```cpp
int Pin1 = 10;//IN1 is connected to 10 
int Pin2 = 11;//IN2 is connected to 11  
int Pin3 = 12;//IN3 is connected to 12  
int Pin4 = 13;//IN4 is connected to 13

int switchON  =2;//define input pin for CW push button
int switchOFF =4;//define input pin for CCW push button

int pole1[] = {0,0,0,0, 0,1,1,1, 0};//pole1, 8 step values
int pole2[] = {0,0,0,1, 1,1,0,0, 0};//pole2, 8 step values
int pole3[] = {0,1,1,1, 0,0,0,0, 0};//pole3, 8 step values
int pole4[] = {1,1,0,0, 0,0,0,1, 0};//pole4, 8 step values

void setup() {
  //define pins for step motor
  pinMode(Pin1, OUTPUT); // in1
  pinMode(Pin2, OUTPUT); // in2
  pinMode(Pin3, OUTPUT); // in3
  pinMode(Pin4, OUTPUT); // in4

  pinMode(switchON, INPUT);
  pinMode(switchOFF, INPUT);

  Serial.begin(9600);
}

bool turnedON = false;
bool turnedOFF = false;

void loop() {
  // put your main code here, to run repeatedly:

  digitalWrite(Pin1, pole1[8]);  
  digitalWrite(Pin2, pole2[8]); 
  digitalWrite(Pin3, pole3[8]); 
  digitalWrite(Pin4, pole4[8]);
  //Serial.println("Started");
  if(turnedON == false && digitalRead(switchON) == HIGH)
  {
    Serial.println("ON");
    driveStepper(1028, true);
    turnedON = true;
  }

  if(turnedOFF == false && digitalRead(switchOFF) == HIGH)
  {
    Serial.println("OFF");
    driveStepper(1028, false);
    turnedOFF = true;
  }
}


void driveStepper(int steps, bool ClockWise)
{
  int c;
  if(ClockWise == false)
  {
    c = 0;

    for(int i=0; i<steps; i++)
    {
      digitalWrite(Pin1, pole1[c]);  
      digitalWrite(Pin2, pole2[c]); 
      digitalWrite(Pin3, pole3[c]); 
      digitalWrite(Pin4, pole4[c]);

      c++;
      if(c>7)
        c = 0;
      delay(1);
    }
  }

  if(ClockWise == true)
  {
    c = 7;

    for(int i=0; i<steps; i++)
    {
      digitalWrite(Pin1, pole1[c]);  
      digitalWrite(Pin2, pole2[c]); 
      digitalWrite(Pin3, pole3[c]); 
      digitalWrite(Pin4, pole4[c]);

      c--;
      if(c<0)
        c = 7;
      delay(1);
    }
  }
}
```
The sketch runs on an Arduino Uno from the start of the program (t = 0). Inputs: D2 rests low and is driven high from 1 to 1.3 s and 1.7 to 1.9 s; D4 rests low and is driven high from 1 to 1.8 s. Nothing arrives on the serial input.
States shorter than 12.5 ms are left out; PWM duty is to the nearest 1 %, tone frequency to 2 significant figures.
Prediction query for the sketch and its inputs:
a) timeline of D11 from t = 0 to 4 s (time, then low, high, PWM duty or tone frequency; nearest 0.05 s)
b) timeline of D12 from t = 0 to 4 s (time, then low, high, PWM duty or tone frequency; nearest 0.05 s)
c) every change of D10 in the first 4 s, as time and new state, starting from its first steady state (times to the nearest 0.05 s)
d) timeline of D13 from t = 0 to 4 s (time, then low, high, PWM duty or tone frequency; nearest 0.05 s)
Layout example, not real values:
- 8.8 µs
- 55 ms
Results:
- 0 s low; 1 s tone 120 Hz; 2.05 s low
- 0 s low; 1 s tone 120 Hz; 2.05 s low
- 0 s low; 1 s tone 120 Hz; 2.05 s low
- 0 s low; 1 s tone 120 Hz; 2.05 s low
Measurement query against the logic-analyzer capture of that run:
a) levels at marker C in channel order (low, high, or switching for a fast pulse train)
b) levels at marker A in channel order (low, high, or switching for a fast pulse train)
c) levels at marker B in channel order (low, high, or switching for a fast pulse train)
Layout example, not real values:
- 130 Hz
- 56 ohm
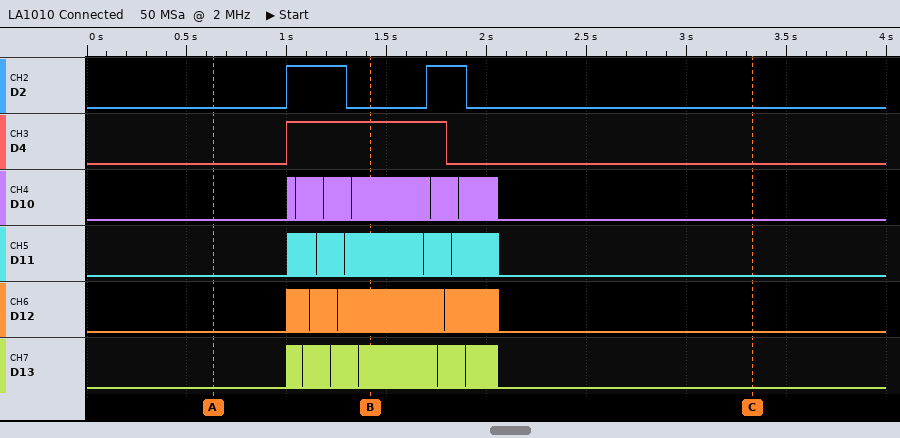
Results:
- D2 low, D4 low, D10 low, D11 low, D12 low, D13 low
- D2 low, D4 low, D10 low, D11 low, D12 low, D13 low
- D2 low, D4 high, D10 switching, D11 switching, D12 switching, D13 switching
